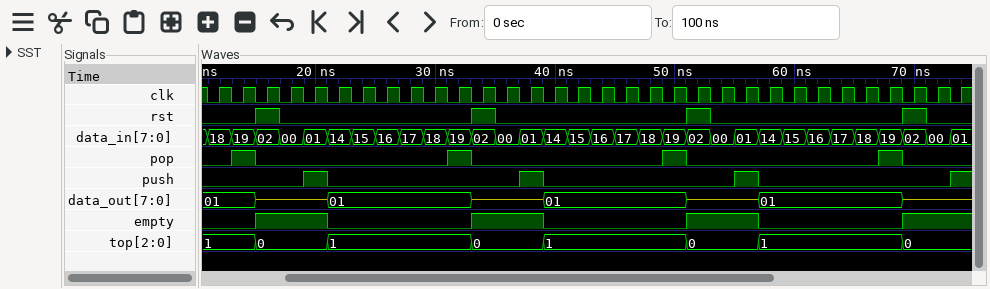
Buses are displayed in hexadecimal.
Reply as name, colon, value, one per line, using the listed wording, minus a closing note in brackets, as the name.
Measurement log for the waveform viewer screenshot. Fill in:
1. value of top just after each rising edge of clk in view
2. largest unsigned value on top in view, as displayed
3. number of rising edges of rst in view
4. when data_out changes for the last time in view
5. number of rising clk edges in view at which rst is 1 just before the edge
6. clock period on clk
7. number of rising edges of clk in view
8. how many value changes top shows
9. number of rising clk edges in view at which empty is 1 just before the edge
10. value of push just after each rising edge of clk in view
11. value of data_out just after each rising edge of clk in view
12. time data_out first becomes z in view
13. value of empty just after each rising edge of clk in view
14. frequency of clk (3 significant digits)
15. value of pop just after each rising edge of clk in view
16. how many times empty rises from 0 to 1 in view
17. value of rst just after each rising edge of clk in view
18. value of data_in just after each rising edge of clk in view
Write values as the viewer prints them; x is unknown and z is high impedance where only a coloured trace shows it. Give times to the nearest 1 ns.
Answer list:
value of top just after each rising edge of clk in view: 1, 1, 0, 0, 0, 1, 1, 1, 1, 1, 1, 0, 0, 0, 1, 1, 1, 1, 1, 1, 0, 0, 0, 1, 1, 1, 1, 1, 1, 0, 0, 0
largest unsigned value on top in view, as displayed: 1
number of rising edges of rst in view: 4
when data_out changes for the last time in view: 69 ns
number of rising clk edges in view at which rst is 1 just before the edge: 4
clock period on clk: 2 ns
number of rising edges of clk in view: 32
how many value changes top shows: 7
number of rising clk edges in view at which empty is 1 just before the edge: 12
value of push just after each rising edge of clk in view: 0 0 0 0 1 0 0 0 0 0 0 0 0 1 0 0 0 0 0 0 0 0 1 0 0 0 0 0 0 0 0 1
value of data_out just after each rising edge of clk in view: 01, 01, z, z, z, 01, 01, 01, 01, 01, 01, z, z, z, 01, 01, 01, 01, 01, 01, z, z, z, 01, 01, 01, 01, 01, 01, z, z, z
time data_out first becomes z in view: 15 ns
value of empty just after each rising edge of clk in view: 0 0 1 1 1 0 0 0 0 0 0 1 1 1 0 0 0 0 0 0 1 1 1 0 0 0 0 0 0 1 1 1
frequency of clk: 500 MHz
value of pop just after each rising edge of clk in view: 0 1 0 0 0 0 0 0 0 0 1 0 0 0 0 0 0 0 0 1 0 0 0 0 0 0 0 0 1 0 0 0
how many times empty rises from 0 to 1 in view: 4
value of rst just after each rising edge of clk in view: 0 0 1 0 0 0 0 0 0 0 0 1 0 0 0 0 0 0 0 0 1 0 0 0 0 0 0 0 0 1 0 0
value of data_in just after each rising edge of clk in view: 18, 19, 02, 00, 01, 14, 15, 16, 17, 18, 19, 02, 00, 01, 14, 15, 16, 17, 18, 19, 02, 00, 01, 14, 15, 16, 17, 18, 19, 02, 00, 01
